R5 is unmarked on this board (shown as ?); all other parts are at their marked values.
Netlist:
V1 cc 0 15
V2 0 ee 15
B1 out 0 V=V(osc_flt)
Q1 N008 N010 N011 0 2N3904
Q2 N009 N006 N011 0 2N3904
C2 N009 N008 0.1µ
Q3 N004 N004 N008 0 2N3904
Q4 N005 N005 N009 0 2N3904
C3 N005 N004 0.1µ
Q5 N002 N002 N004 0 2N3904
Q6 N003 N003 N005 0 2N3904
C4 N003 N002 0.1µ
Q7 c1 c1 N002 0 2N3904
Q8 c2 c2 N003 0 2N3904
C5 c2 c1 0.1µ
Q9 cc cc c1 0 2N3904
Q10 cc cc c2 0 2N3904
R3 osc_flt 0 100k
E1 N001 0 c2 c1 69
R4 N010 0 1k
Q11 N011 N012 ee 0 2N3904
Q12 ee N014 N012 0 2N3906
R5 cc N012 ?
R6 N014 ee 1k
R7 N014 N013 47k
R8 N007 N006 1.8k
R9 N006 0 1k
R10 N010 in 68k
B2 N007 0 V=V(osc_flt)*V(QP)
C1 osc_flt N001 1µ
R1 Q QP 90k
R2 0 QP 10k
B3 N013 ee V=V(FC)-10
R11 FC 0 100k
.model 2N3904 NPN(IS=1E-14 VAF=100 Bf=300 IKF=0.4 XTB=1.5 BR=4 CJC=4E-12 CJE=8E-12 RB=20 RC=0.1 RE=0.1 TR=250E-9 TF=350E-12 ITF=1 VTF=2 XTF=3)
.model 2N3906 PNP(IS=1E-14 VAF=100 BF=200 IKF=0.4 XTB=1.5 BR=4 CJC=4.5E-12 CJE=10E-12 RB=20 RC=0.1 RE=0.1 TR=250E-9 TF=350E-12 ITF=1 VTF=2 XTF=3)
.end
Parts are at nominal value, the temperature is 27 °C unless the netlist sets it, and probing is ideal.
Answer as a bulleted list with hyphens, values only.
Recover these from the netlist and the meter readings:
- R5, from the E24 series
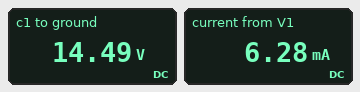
- 4.7 kΩ
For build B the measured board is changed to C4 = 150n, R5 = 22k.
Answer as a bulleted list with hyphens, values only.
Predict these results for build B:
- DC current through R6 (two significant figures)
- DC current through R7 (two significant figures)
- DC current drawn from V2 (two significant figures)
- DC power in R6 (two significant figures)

- 200 µA
- 210 µA
- 1.3 mA
- 41 µW
